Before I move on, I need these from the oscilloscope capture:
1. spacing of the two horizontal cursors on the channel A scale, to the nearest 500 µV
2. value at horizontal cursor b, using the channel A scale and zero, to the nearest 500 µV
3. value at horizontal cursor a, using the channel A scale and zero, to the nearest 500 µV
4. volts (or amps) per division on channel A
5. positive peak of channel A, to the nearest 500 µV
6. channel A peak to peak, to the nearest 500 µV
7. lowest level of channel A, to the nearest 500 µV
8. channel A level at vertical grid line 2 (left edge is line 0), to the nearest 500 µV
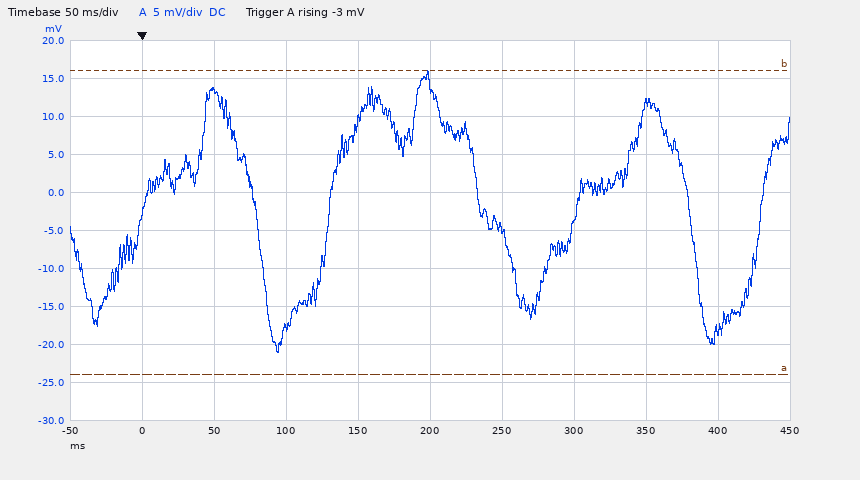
40.0 mV
16.0 mV
-24.0 mV
5 mV
16.0 mV
37.0 mV
-21.0 mV
13.5 mV
